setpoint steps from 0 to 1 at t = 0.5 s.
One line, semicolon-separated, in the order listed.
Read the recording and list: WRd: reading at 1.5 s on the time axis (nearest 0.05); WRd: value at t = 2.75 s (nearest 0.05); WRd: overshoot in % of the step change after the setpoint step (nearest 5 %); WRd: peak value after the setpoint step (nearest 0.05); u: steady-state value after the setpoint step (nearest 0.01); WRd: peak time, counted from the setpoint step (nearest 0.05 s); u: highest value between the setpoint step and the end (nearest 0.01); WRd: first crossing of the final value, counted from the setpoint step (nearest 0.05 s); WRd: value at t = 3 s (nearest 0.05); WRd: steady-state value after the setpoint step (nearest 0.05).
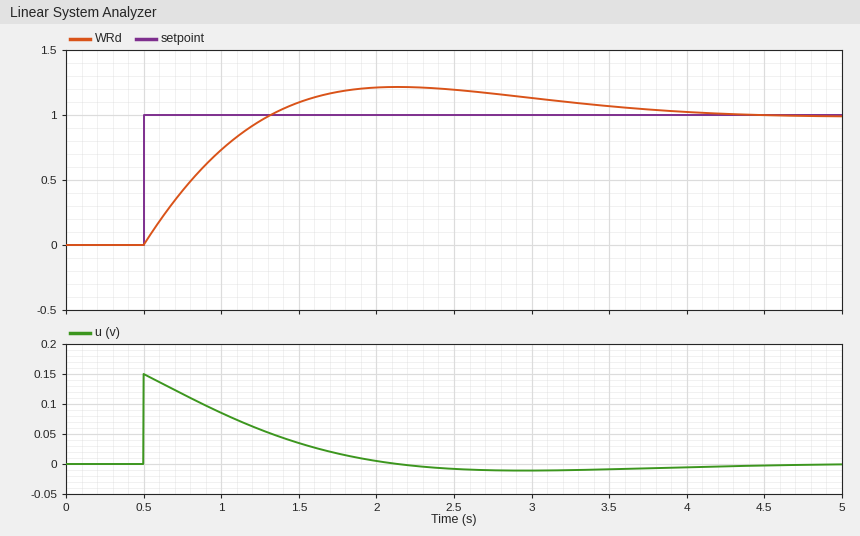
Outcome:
1.10; 1.15; 20 %; 1.20; 0.00; 1.65 s; 0.15; 0.80 s; 1.15; 1.00
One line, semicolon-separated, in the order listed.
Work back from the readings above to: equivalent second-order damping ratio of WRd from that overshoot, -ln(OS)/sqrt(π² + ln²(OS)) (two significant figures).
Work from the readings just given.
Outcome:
0.46
